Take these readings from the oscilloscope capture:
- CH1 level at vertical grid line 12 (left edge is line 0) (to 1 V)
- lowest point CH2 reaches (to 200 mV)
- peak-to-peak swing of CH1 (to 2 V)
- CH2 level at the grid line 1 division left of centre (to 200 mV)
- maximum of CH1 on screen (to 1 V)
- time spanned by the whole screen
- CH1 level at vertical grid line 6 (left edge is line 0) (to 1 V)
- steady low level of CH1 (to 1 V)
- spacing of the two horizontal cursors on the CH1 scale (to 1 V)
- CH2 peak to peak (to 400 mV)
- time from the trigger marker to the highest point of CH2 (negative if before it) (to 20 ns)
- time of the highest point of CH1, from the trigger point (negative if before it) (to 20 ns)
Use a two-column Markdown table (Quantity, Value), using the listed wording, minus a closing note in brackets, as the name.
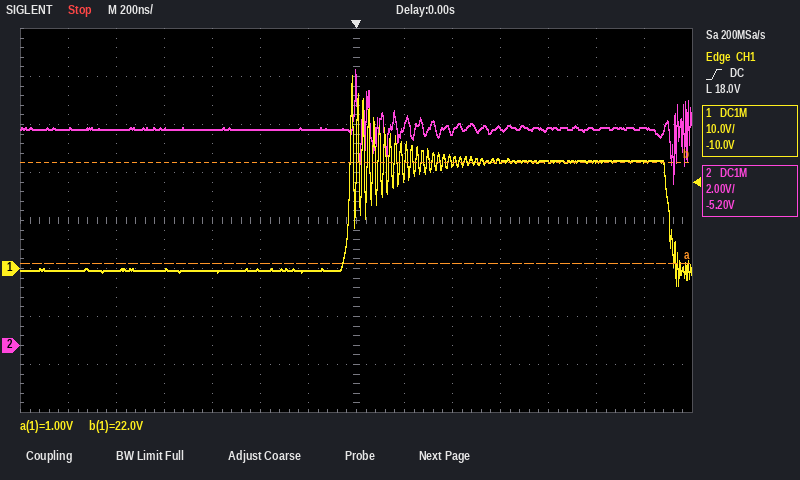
| Quantity | Value |
|---|---|
| CH1 level at vertical grid line 12 (left edge is line 0) | 22 V |
| lowest point CH2 reaches | 6.8 V |
| peak-to-peak swing of CH1 | 44 V |
| CH2 level at the grid line 1 division left of centre | 9.0 V |
| maximum of CH1 on screen | 40 V |
| time spanned by the whole screen | 2.8 µs |
| CH1 level at vertical grid line 6 (left edge is line 0) | 0 V |
| steady low level of CH1 | 0 V |
| spacing of the two horizontal cursors on the CH1 scale | 21 V |
| CH2 peak to peak | 4.8 V |
| time from the trigger marker to the highest point of CH2 (negative if before it) | 0 ns |
| time of the highest point of CH1, from the trigger point (negative if before it) | -20 ns |
